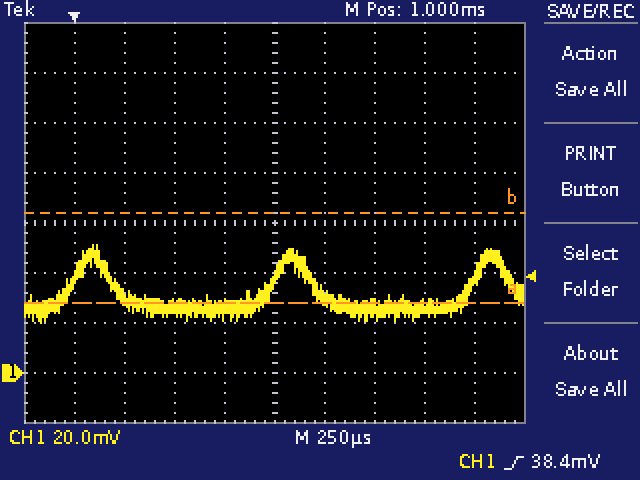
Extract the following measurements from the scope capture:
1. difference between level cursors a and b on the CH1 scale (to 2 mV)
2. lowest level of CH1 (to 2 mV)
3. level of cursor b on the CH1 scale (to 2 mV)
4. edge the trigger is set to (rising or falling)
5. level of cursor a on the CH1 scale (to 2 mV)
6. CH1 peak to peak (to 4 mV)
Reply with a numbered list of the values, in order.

1. 36 mV
2. 20 mV
3. 64 mV
4. rising
5. 28 mV
6. 32 mV
